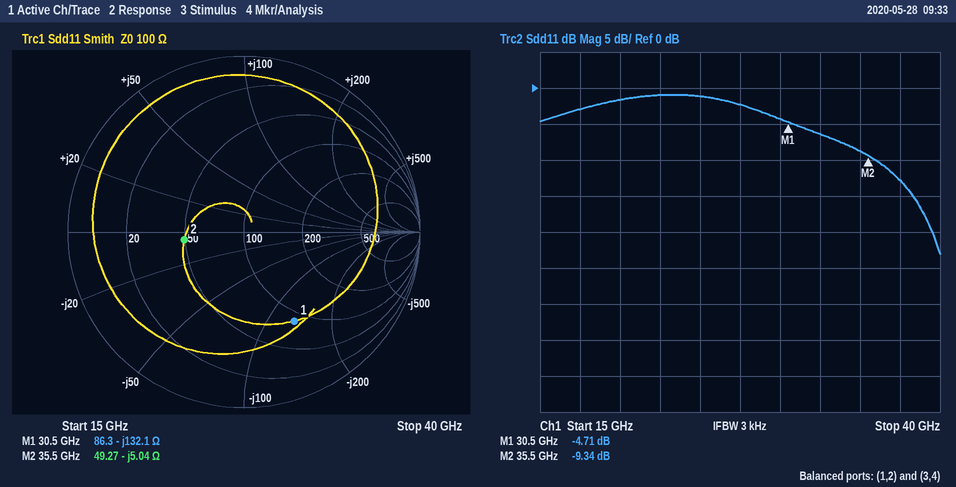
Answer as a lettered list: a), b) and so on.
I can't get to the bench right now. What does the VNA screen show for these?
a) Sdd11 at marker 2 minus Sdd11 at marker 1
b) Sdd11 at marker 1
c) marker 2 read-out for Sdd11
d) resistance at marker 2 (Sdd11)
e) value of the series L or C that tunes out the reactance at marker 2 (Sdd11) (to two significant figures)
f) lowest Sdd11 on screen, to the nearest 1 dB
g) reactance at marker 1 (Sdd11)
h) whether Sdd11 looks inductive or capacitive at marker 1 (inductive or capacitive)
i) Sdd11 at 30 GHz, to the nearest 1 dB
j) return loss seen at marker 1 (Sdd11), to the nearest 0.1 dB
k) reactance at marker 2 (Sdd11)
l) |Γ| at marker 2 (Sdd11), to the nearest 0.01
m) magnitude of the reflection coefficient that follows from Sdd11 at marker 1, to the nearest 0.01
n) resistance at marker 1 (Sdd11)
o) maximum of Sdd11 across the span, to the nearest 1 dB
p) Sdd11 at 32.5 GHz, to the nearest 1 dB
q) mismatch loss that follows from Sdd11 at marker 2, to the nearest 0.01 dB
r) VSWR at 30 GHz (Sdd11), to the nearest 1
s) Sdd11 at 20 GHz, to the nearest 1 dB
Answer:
a) -4.63 dB
b) -4.71 dB
c) -9.34 dB
d) 49.27 Ω
e) 23 pH
f) -23 dB
g) -132.1 Ω
h) capacitive
i) -4 dB
j) 4.7 dB
k) -5.04 Ω
l) 0.34
m) 0.58
n) 86.3 Ω
o) -1 dB
p) -6 dB
q) 0.54 dB
r) 4
s) -2 dB
